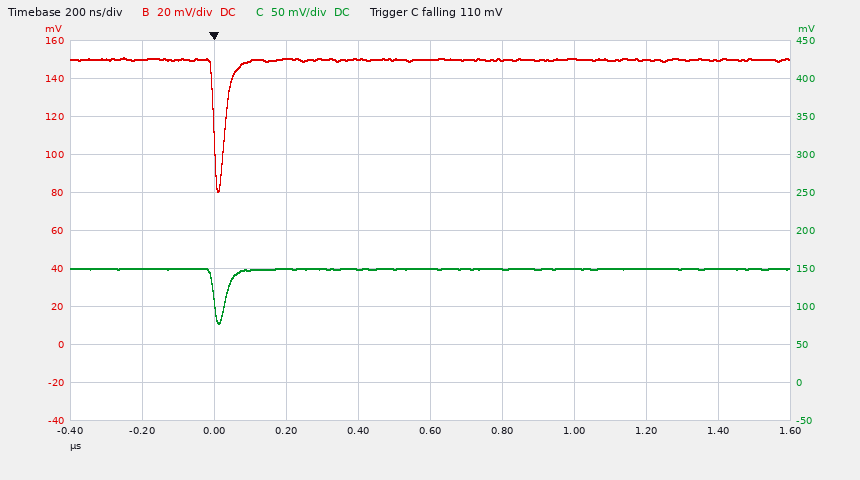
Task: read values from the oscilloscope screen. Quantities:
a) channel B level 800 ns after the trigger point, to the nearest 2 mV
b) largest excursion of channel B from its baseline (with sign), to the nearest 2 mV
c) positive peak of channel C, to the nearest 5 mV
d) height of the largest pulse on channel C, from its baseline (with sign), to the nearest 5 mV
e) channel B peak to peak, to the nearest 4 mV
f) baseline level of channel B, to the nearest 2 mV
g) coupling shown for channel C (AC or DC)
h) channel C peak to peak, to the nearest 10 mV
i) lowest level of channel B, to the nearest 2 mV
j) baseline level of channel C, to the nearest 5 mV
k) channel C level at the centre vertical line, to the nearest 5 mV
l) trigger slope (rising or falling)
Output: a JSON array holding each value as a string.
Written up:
["150 mV", "-70 mV", "150 mV", "-70 mV", "72 mV", "150 mV", "DC", "70 mV", "80 mV", "150 mV", "150 mV", "falling"]
